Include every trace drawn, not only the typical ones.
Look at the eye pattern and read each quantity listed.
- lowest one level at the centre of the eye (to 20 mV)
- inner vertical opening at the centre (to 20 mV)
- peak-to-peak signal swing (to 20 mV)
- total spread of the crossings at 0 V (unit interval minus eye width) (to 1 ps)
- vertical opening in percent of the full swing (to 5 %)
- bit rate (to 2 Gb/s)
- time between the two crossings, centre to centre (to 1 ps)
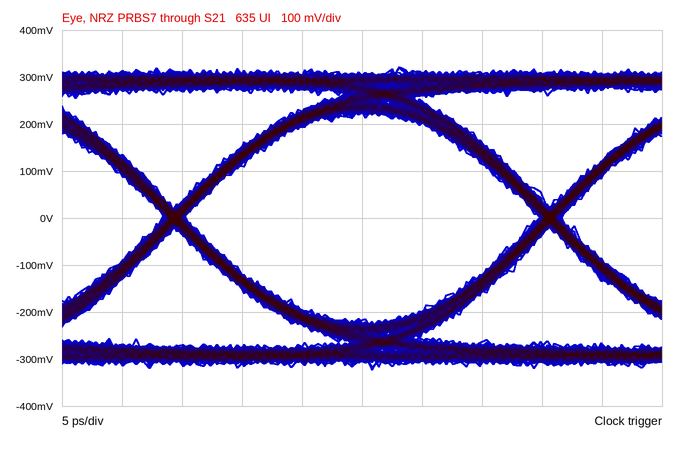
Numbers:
220 mV
440 mV
640 mV
2 ps
70 %
32 Gb/s
31 ps
